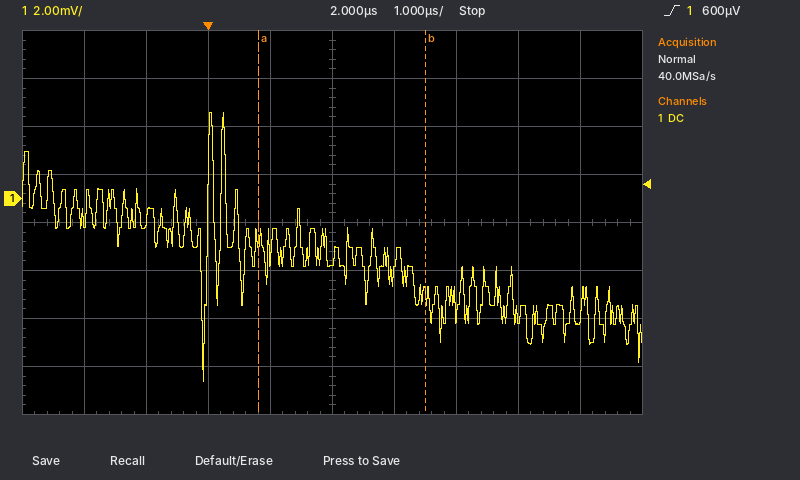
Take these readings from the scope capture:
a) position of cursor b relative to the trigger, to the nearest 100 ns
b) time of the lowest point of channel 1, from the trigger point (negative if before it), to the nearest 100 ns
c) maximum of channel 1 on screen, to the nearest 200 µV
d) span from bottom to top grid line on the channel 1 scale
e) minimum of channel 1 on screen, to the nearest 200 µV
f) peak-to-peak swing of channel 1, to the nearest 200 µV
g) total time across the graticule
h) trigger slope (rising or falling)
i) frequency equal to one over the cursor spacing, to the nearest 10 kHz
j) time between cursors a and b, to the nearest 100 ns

+3.5 µs
-100 ns
3.6 mV
16 mV
-7.6 mV
11.2 mV
10 µs
rising
370 kHz
2.7 µs
